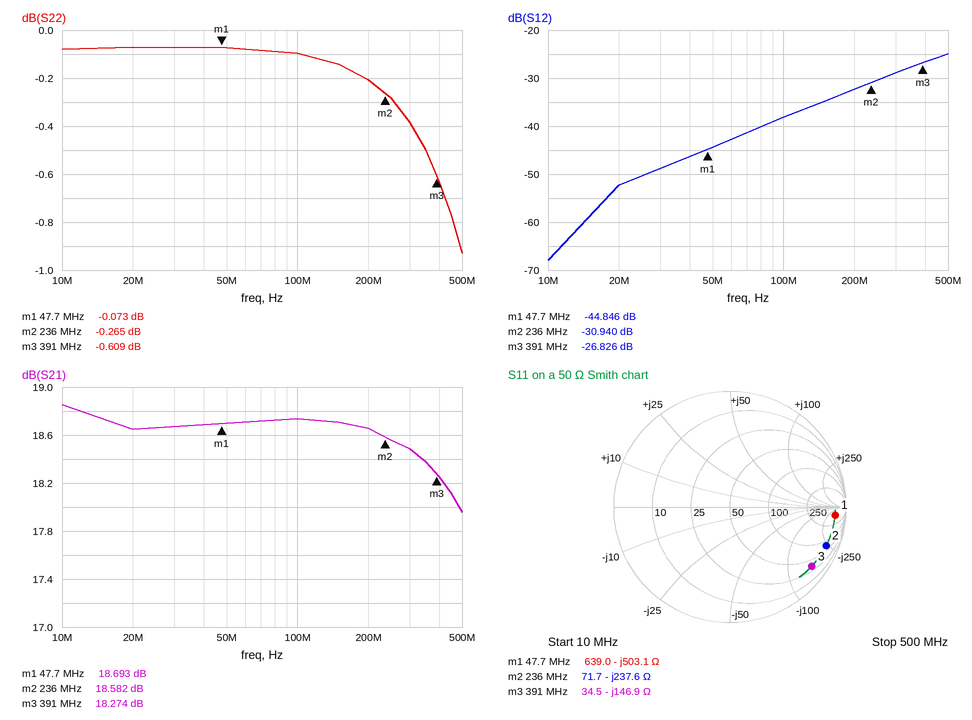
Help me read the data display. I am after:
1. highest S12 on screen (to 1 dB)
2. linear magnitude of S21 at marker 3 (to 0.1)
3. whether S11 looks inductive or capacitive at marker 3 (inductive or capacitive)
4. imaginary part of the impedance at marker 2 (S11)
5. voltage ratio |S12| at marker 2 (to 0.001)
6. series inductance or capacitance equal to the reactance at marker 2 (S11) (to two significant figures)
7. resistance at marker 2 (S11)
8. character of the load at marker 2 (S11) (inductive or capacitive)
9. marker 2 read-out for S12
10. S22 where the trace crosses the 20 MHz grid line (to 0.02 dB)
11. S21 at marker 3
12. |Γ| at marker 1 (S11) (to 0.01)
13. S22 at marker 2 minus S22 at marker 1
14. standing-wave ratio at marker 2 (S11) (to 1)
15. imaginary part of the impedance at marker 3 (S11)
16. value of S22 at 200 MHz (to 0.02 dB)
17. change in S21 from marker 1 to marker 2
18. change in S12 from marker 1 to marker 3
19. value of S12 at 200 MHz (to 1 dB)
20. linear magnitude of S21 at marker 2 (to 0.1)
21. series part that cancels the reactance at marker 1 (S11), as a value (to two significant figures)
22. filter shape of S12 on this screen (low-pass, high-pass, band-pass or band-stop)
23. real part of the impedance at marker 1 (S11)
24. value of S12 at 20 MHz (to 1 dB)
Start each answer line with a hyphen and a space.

- -25 dB
- 8.2
- capacitive
- -237.6 Ω
- 0.028
- 2.8 pF
- 71.7 Ω
- capacitive
- -30.940 dB
- -0.08 dB
- 18.274 dB
- 0.91
- -0.192 dB
- 18
- -146.9 Ω
- -0.20 dB
- -0.111 dB
- 18.020 dB
- -32 dB
- 8.5
- 1.7 µH
- high-pass
- 639.0 Ω
- -52 dB
